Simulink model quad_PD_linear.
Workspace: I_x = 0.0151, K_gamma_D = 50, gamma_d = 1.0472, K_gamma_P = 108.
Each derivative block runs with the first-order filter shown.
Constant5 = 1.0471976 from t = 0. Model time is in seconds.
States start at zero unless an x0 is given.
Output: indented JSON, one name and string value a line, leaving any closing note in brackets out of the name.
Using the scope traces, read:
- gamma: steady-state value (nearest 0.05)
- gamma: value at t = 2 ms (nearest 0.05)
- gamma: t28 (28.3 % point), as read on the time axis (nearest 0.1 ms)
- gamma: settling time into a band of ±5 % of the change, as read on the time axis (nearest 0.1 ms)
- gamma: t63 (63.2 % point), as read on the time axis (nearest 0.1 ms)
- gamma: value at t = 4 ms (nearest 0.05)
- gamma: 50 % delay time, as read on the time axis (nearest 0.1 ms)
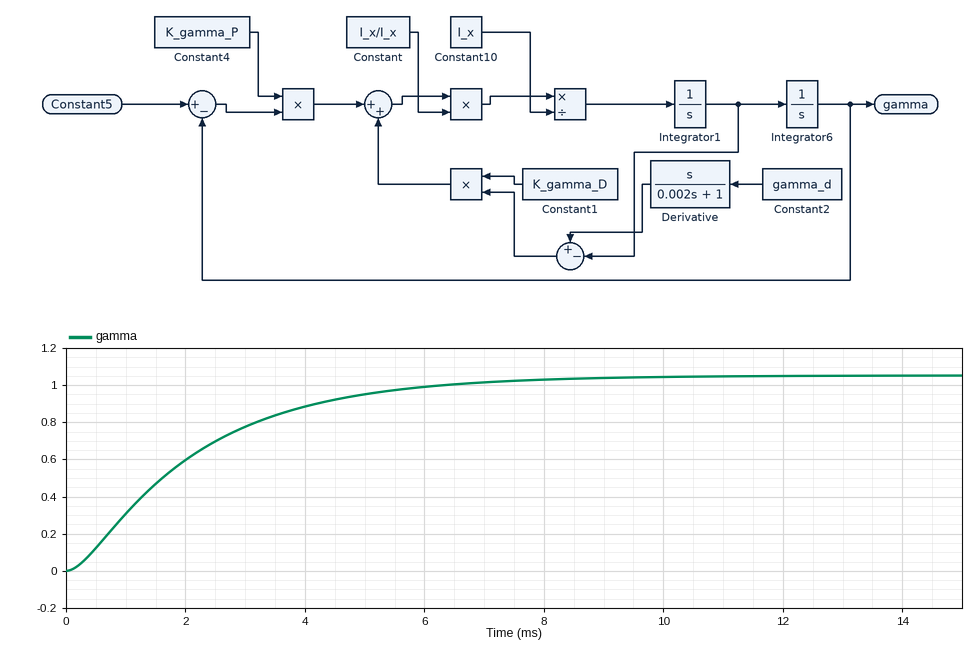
{
  "gamma: steady-state value": "1.05",
  "gamma: value at t = 2 ms": "0.60",
  "gamma: t28 (28.3 % point), as read on the time axis": "1.0 ms",
  "gamma: settling time into a band of ±5 % of the change, as read on the time axis": "6.3 ms",
  "gamma: t63 (63.2 % point), as read on the time axis": "2.3 ms",
  "gamma: value at t = 4 ms": "0.90",
  "gamma: 50 % delay time, as read on the time axis": "1.7 ms"
}
